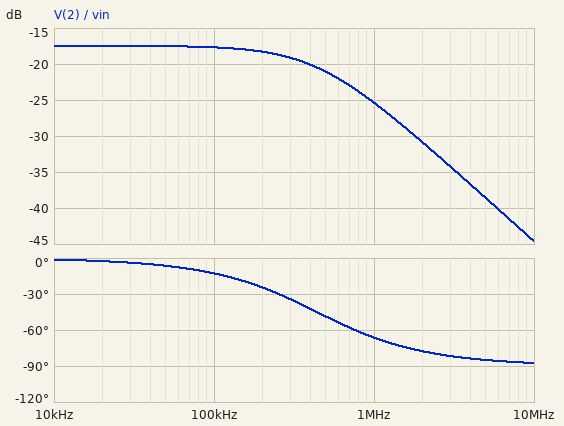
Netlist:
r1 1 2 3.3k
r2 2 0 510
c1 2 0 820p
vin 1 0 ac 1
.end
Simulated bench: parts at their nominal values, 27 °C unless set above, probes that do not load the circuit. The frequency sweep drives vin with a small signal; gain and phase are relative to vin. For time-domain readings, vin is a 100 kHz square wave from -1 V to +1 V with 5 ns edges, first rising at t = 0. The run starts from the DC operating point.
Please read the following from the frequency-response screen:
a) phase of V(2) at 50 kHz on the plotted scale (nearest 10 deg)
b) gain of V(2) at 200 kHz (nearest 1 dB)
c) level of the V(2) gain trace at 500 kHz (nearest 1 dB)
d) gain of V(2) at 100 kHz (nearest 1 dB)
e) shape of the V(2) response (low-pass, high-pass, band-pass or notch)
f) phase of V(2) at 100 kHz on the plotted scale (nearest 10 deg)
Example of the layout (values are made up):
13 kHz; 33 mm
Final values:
-10 deg; -18 dB; -21 dB; -18 dB; low-pass; -10 deg
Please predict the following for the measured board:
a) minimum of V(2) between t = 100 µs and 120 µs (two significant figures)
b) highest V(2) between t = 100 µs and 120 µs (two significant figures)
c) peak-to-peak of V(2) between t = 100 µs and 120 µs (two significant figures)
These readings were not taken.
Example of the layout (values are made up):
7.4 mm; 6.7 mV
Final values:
-130 mV; 130 mV; 270 mV
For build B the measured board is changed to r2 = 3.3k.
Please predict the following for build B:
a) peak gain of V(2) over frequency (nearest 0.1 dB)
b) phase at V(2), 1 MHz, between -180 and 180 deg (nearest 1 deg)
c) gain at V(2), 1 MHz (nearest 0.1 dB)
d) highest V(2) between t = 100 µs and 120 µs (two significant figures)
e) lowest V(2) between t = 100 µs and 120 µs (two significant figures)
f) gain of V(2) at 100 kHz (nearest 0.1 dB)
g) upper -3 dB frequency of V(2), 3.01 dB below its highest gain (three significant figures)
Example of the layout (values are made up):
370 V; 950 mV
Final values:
-6.0 dB; -83 deg; -24.7 dB; 480 mV; -480 mV; -8.4 dB; 118 kHz
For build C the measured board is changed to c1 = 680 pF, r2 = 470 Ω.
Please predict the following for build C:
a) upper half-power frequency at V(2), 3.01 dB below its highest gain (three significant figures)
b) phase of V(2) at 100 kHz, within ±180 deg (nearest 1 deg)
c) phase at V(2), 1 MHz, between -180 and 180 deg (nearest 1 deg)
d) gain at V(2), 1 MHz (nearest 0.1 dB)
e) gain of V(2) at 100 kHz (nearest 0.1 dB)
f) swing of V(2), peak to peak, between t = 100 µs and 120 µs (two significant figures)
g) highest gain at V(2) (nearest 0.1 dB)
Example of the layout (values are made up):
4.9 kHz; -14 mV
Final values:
569 kHz; -10 deg; -60 deg; -24.2 dB; -18.2 dB; 250 mV; -18.1 dB
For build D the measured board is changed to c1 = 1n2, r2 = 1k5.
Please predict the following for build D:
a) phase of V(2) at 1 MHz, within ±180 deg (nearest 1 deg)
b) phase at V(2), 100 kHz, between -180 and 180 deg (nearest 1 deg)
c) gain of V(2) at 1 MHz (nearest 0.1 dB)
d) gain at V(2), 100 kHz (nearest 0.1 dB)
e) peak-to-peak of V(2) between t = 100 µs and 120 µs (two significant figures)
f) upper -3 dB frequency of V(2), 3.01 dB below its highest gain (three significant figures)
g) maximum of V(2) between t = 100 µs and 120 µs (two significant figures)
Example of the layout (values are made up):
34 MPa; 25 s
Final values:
-83 deg; -38 deg; -28.0 dB; -12.2 dB; 600 mV; 129 kHz; 300 mV
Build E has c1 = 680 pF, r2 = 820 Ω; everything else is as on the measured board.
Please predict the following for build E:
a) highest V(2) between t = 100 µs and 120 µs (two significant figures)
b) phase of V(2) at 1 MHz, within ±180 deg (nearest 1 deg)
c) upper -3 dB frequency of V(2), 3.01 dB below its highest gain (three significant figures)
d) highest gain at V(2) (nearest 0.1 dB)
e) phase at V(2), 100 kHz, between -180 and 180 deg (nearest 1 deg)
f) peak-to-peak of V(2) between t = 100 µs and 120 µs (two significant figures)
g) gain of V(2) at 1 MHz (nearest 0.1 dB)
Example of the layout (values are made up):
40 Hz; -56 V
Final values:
200 mV; -70 deg; 356 kHz; -14.0 dB; -16 deg; 400 mV; -23.5 dB
